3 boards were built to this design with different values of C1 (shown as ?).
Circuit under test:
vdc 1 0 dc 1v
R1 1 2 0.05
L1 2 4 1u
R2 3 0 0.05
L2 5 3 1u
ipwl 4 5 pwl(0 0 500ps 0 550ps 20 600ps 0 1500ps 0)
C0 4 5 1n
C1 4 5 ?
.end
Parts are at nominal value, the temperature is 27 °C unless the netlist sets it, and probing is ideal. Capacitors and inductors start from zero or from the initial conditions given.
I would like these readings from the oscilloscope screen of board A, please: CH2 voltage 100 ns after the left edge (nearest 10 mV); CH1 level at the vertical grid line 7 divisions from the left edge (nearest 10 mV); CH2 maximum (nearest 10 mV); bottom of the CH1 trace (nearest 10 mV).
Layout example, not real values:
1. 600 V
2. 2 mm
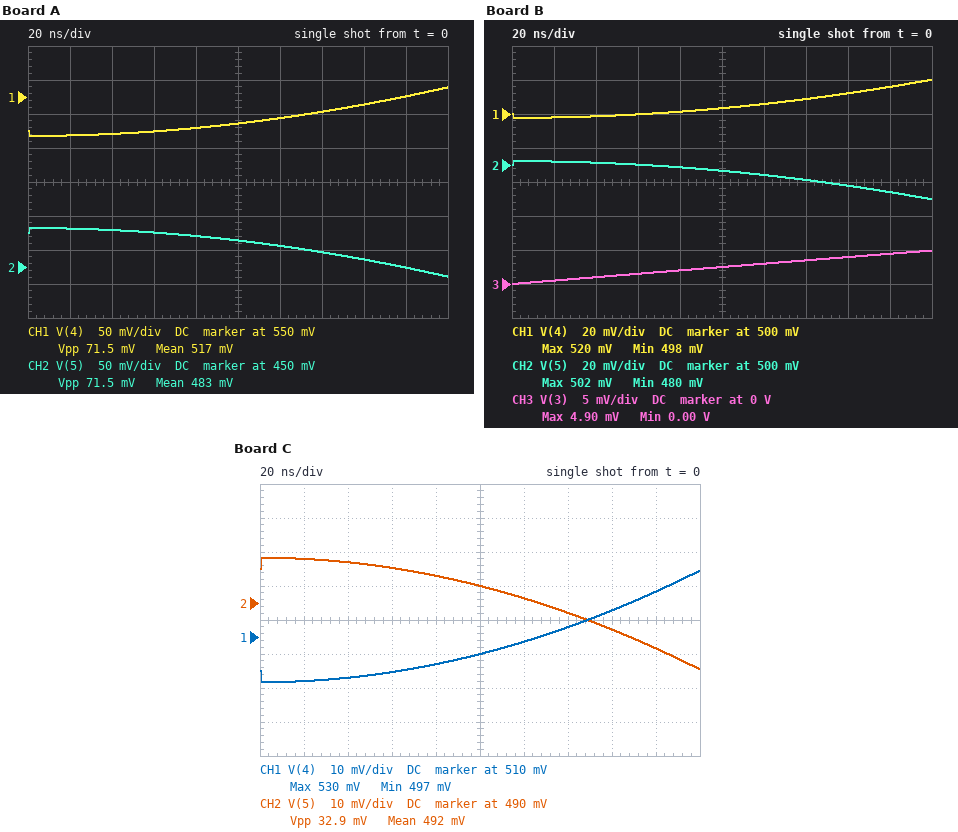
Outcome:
1. 490 mV
2. 530 mV
3. 510 mV
4. 490 mV
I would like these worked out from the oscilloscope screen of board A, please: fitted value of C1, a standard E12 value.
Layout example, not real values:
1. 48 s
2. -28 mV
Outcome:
1. 68 nF
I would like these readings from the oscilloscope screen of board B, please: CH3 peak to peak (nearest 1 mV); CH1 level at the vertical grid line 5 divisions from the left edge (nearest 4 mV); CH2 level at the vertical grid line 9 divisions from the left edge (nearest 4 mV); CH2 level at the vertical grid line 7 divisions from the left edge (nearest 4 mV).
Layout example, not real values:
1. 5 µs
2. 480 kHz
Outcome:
1. 5 mV
2. 504 mV
3. 484 mV
4. 492 mV
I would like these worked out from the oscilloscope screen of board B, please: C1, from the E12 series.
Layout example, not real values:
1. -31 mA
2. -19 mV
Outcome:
1. 220 nF
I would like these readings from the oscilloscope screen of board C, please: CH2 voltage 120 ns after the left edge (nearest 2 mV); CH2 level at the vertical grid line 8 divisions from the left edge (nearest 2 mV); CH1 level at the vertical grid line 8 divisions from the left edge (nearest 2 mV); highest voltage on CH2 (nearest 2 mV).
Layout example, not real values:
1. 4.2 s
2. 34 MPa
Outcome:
1. 492 mV
2. 482 mV
3. 518 mV
4. 504 mV
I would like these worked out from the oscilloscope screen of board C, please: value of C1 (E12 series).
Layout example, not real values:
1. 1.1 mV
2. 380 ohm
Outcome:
1. 150 nF
